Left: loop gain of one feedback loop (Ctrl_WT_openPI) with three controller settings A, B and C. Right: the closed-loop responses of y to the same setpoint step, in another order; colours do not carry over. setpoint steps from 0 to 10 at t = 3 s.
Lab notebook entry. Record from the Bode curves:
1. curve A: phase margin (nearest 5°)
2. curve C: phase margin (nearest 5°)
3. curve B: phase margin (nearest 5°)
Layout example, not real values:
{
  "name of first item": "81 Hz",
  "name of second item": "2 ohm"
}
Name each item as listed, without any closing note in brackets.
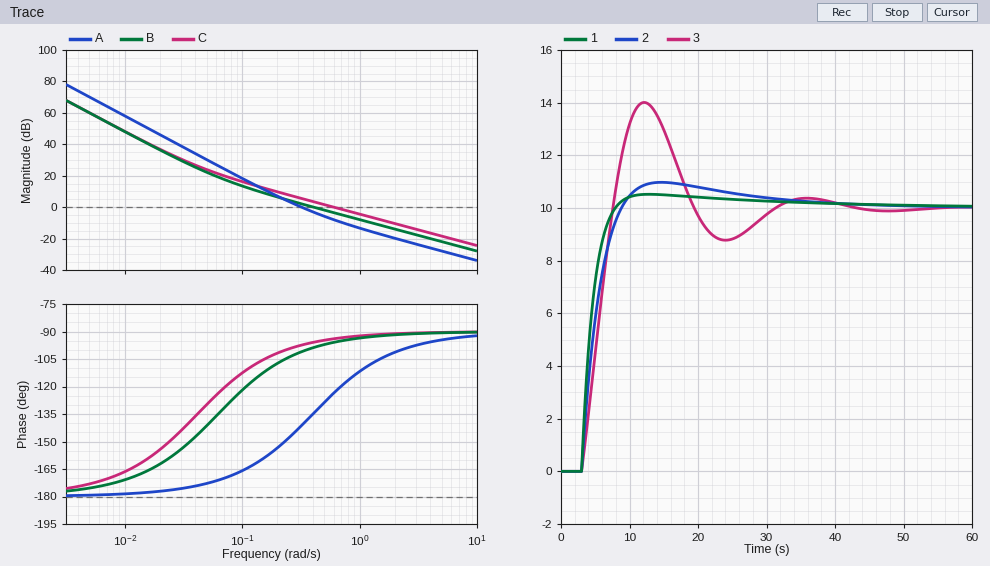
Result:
{
  "curve A: phase margin": "40°",
  "curve C: phase margin": "85°",
  "curve B: phase margin": "80°"
}
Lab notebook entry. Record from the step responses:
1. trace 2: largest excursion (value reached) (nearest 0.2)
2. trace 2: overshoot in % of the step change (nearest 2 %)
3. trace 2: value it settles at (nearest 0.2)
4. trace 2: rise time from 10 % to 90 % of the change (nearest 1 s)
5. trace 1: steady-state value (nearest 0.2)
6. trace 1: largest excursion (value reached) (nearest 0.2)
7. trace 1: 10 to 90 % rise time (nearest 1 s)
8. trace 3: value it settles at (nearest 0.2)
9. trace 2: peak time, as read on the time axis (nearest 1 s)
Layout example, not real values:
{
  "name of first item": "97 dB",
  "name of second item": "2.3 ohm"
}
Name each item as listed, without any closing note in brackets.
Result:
{
  "trace 2: largest excursion (value reached)": "11.0",
  "trace 2: overshoot in % of the step change": "10 %",
  "trace 2: value it settles at": "10.0",
  "trace 2: rise time from 10 % to 90 % of the change": "4 s",
  "trace 1: steady-state value": "10.0",
  "trace 1: largest excursion (value reached)": "10.6",
  "trace 1: 10 to 90 % rise time": "3 s",
  "trace 3: value it settles at": "10.0",
  "trace 2: peak time, as read on the time axis": "15 s"
}
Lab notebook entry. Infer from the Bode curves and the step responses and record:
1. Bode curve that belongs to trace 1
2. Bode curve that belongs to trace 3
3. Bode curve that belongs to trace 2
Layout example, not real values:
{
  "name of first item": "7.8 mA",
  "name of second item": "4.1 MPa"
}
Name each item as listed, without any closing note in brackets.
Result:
{
  "Bode curve that belongs to trace 1": "C",
  "Bode curve that belongs to trace 3": "A",
  "Bode curve that belongs to trace 2": "B"
}
